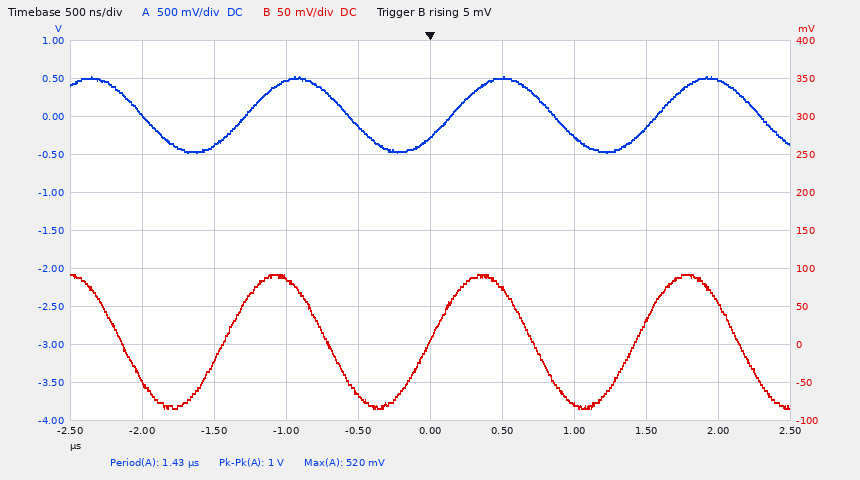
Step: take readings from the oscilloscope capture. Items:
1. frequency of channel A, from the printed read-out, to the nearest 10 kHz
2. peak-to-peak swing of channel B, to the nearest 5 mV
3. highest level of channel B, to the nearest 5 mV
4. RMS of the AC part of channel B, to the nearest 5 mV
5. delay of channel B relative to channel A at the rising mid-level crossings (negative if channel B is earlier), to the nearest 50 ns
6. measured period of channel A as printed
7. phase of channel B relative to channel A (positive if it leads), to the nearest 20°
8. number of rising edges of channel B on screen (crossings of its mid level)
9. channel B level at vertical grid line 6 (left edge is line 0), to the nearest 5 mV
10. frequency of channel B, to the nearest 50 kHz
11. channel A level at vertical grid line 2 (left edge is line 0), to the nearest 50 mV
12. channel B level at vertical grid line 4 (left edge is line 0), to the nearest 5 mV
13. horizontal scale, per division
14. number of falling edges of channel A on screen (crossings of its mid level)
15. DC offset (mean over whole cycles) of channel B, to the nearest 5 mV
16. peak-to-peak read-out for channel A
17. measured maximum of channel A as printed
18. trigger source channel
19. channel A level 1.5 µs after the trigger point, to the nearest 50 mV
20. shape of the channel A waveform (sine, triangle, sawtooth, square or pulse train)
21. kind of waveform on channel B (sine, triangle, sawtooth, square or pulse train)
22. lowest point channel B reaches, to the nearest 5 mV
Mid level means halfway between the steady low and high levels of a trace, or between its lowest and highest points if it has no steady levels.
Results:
700 kHz
175 mV
90 mV
60 mV
-150 ns
1.43 µs
+40°
3
75 mV
700 kHz
-400 mV
-65 mV
500 ns
4
5 mV
1 V
520 mV
channel B
-150 mV
sine
sine
-85 mV
